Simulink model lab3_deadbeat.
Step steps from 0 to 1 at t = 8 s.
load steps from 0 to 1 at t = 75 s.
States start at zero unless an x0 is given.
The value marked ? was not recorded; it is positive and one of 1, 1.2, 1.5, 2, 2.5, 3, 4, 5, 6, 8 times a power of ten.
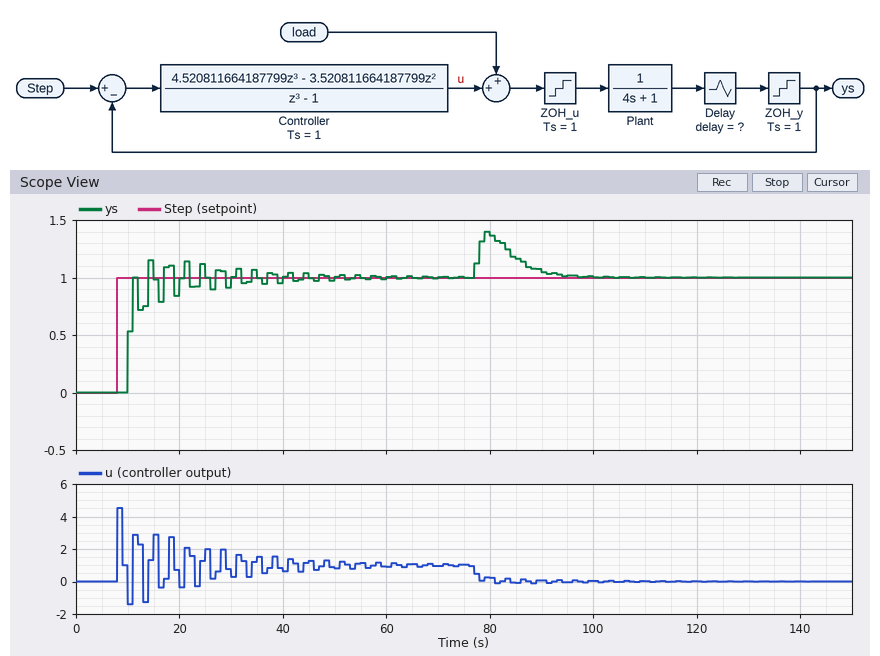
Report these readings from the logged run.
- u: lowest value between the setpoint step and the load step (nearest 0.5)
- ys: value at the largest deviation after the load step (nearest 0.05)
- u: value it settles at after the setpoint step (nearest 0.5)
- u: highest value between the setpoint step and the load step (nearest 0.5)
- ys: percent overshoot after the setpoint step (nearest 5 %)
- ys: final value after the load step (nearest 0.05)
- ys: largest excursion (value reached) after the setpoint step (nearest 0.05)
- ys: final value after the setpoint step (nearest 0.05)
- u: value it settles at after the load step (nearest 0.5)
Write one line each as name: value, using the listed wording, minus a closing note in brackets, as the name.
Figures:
u: lowest value between the setpoint step and the load step: -1.5
ys: value at the largest deviation after the load step: 1.40
u: value it settles at after the setpoint step: 1.0
u: highest value between the setpoint step and the load step: 4.5
ys: percent overshoot after the setpoint step: 15 %
ys: final value after the load step: 1.00
ys: largest excursion (value reached) after the setpoint step: 1.15
ys: final value after the setpoint step: 1.00
u: value it settles at after the load step: 0.0
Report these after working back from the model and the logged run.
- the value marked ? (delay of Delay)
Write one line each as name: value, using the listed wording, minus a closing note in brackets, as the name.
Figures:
the value marked ?: 1.5
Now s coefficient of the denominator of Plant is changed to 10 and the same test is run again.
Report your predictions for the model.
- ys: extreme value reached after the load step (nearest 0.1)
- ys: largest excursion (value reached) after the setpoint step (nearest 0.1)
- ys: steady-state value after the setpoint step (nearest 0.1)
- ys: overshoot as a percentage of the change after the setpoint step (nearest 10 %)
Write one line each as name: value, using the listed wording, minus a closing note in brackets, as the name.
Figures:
ys: extreme value reached after the load step: 1.3
ys: largest excursion (value reached) after the setpoint step: 1.2
ys: steady-state value after the setpoint step: 1.0
ys: overshoot as a percentage of the change after the setpoint step: 20 %
